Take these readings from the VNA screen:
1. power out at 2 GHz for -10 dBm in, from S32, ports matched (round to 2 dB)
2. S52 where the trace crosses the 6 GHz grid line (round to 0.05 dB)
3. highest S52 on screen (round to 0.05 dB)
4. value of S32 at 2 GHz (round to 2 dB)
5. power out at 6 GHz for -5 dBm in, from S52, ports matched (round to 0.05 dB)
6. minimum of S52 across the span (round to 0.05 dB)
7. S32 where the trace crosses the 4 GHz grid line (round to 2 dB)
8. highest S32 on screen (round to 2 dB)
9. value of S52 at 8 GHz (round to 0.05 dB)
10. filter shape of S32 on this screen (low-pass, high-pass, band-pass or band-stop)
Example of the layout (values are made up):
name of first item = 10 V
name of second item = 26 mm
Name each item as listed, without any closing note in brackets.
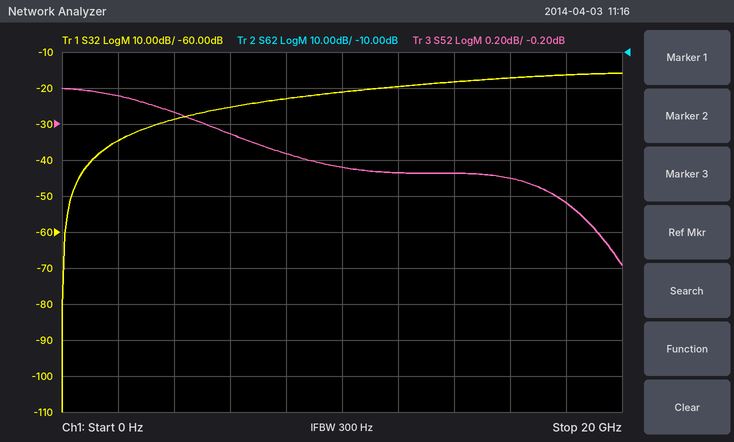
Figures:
power out at 2 GHz for -10 dBm in, from S32, ports matched = -44 dBm
S52 where the trace crosses the 6 GHz grid line = -0.25 dB
highest S52 on screen = 0.00 dB
value of S32 at 2 GHz = -34 dB
power out at 6 GHz for -5 dBm in, from S52, ports matched = -5.25 dBm
minimum of S52 across the span = -1.00 dB
S32 where the trace crosses the 4 GHz grid line = -28 dB
highest S32 on screen = -16 dB
value of S52 at 8 GHz = -0.35 dB
filter shape of S32 on this screen = high-pass
